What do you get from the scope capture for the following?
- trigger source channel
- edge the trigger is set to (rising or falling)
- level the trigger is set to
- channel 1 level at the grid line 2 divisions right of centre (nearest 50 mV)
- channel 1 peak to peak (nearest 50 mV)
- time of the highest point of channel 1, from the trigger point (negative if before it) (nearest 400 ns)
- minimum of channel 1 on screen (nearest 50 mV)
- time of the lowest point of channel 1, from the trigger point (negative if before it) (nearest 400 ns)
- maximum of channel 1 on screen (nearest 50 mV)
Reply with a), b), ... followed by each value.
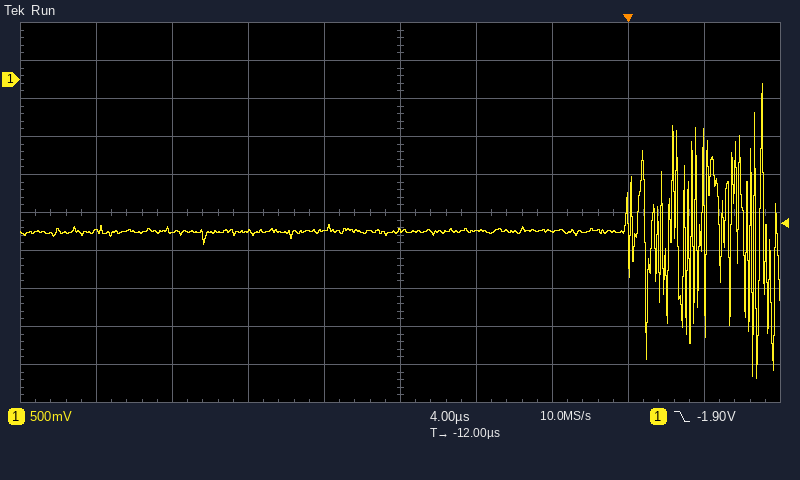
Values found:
a) channel 1
b) falling
c) -1.90 V
d) -2.00 V
e) 3.90 V
f) +7.2 µs
g) -3.95 V
h) +6.8 µs
i) -50 mV
